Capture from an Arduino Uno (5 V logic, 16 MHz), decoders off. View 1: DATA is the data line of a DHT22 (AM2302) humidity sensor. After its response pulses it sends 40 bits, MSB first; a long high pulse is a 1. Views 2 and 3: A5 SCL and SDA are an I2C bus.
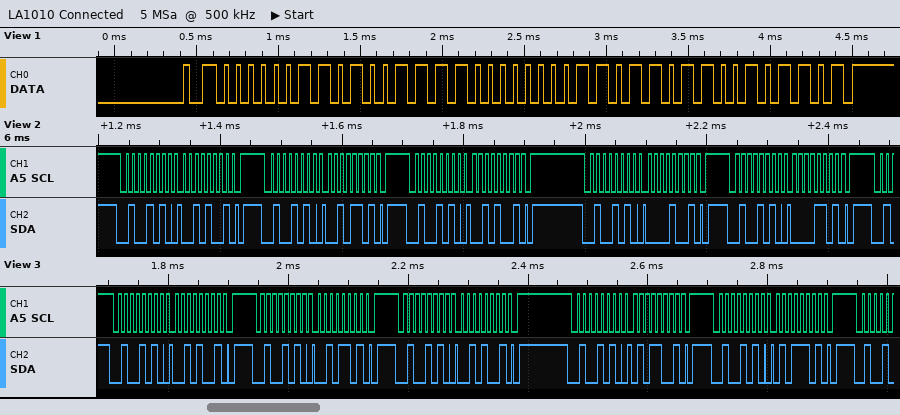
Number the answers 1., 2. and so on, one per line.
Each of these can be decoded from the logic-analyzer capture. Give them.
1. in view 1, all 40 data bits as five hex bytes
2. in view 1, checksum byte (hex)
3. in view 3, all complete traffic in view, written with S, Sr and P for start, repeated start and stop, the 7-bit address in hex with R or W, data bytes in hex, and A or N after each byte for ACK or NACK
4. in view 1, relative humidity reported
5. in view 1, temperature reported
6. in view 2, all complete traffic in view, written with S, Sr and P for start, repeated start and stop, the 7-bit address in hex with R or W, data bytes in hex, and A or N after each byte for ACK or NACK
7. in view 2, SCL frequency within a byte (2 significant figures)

1. 03 4F 00 DB 2D
2. 0x2D
3. S 25W A 29 A P S 25W A 2D A P S 25W A 29 A P S 25W A 59 A P S 25W A 5D A P
4. 84.7 %
5. 21.9 °C
6. S 25W A 29 A P S 25W A 2D A P S 25W A 29 A P S 25W A 09 A P S 25W A 0D A P
7. 100 kHz
